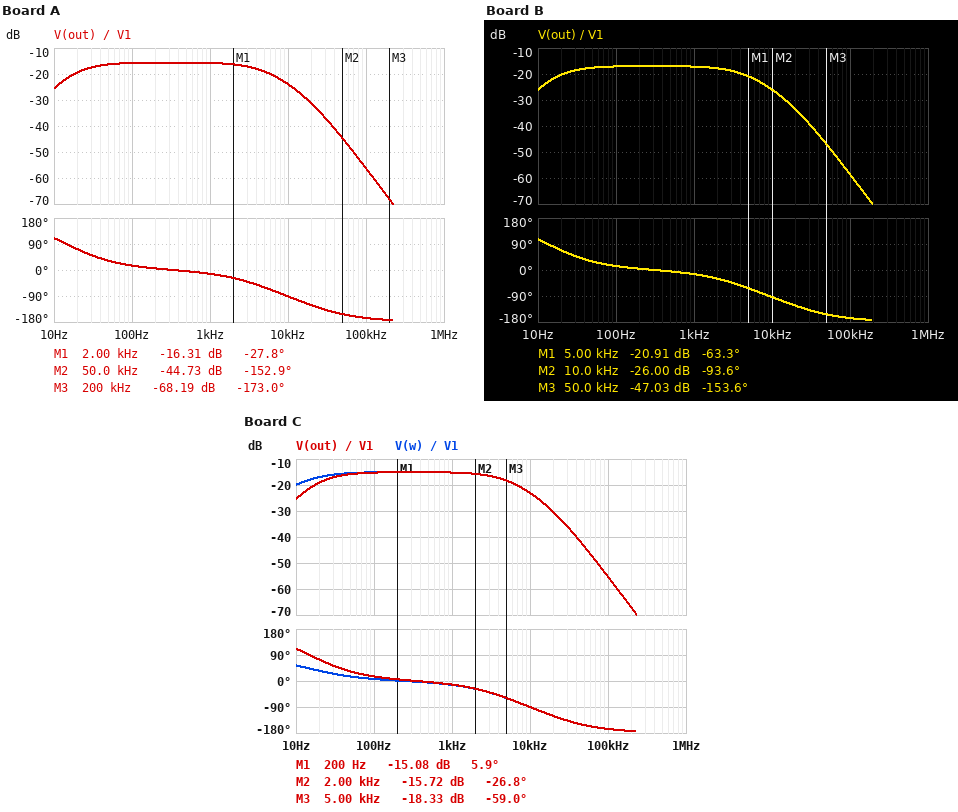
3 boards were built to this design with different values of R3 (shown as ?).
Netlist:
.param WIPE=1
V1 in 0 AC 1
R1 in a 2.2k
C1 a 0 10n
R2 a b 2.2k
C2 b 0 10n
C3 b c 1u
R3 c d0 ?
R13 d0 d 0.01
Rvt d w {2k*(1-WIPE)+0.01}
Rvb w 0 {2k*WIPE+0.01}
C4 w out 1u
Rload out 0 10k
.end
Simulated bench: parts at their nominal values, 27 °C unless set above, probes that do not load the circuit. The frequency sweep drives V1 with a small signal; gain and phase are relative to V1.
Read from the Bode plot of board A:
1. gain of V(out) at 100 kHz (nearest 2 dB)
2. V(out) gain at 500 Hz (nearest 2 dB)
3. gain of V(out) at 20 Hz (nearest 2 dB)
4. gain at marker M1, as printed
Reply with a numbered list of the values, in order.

1. -56 dB
2. -16 dB
3. -20 dB
4. -16.31 dB
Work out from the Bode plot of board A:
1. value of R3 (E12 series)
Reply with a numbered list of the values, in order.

1. 3.9 kΩ
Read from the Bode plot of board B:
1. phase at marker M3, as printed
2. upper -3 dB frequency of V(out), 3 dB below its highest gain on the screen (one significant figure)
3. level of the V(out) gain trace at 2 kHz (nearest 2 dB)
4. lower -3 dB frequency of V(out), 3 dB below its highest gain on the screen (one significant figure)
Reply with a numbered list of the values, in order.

1. -153.6 deg
2. 4 kHz
3. -18 dB
4. 20 Hz
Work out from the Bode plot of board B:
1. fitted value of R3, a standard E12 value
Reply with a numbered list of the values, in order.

1. 5.6 kΩ
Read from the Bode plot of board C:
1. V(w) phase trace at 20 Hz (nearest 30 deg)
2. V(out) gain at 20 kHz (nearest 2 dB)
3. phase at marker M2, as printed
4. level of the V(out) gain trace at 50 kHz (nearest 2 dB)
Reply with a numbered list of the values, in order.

1. 30 deg
2. -30 dB
3. -26.8 deg
4. -44 dB
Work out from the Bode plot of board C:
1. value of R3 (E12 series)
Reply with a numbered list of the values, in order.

1. 3.3 kΩ
